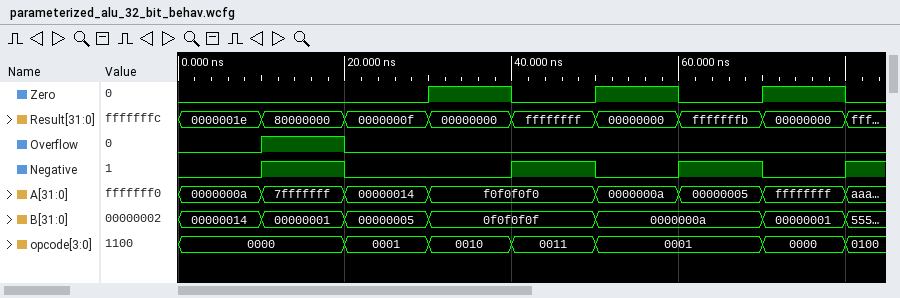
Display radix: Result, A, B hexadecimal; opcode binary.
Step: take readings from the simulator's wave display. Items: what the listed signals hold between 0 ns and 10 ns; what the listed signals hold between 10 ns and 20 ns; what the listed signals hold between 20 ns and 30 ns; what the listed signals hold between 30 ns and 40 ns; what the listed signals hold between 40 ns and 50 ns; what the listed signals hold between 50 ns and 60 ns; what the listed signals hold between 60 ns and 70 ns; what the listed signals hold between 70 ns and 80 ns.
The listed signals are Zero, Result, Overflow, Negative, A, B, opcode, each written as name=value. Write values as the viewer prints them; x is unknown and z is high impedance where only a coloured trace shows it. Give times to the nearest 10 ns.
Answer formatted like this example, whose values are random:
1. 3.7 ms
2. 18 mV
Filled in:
1. Zero=0, Result=0000001e, Overflow=0, Negative=0, A=0000000a, B=00000014, opcode=0000
2. Zero=0, Result=80000000, Overflow=1, Negative=1, A=7fffffff, B=00000001, opcode=0000
3. Zero=0, Result=0000000f, Overflow=0, Negative=0, A=00000014, B=00000005, opcode=0001
4. Zero=1, Result=00000000, Overflow=0, Negative=0, A=f0f0f0f0, B=0f0f0f0f, opcode=0010
5. Zero=0, Result=ffffffff, Overflow=0, Negative=1, A=f0f0f0f0, B=0f0f0f0f, opcode=0011
6. Zero=1, Result=00000000, Overflow=0, Negative=0, A=0000000a, B=0000000a, opcode=0001
7. Zero=0, Result=fffffffb, Overflow=0, Negative=1, A=00000005, B=0000000a, opcode=0001
8. Zero=1, Result=00000000, Overflow=0, Negative=0, A=ffffffff, B=00000001, opcode=0000
